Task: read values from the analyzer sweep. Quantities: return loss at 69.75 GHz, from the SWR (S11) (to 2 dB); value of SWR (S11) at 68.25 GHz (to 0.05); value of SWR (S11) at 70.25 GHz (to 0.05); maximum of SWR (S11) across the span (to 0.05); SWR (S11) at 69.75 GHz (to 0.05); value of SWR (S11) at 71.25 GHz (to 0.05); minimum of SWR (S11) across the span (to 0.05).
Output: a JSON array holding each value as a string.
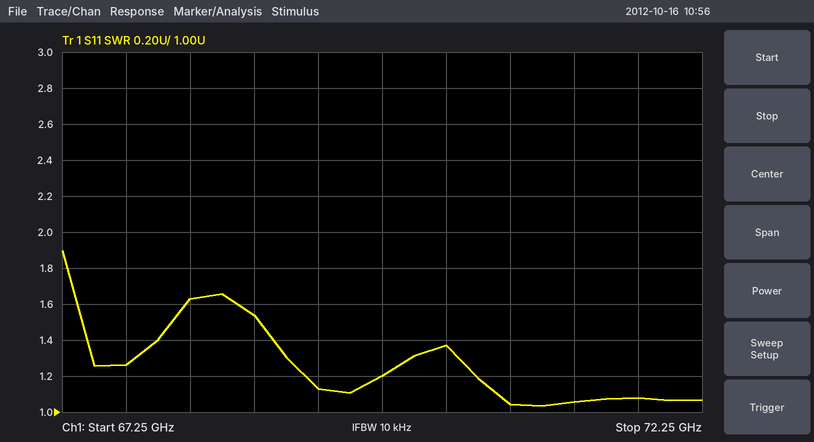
["20 dB", "1.65", "1.35", "1.90", "1.20", "1.05", "1.05"]
